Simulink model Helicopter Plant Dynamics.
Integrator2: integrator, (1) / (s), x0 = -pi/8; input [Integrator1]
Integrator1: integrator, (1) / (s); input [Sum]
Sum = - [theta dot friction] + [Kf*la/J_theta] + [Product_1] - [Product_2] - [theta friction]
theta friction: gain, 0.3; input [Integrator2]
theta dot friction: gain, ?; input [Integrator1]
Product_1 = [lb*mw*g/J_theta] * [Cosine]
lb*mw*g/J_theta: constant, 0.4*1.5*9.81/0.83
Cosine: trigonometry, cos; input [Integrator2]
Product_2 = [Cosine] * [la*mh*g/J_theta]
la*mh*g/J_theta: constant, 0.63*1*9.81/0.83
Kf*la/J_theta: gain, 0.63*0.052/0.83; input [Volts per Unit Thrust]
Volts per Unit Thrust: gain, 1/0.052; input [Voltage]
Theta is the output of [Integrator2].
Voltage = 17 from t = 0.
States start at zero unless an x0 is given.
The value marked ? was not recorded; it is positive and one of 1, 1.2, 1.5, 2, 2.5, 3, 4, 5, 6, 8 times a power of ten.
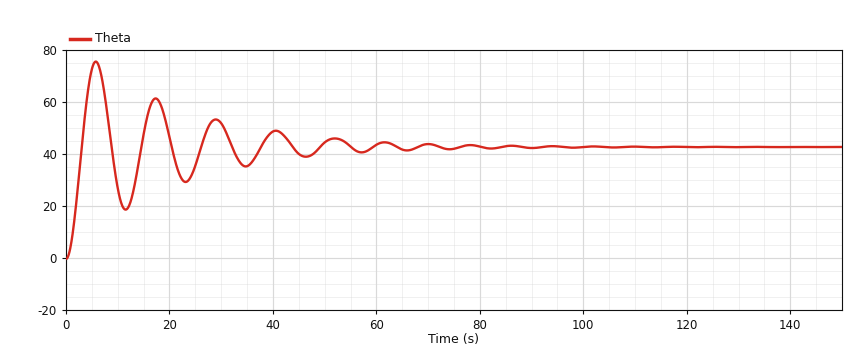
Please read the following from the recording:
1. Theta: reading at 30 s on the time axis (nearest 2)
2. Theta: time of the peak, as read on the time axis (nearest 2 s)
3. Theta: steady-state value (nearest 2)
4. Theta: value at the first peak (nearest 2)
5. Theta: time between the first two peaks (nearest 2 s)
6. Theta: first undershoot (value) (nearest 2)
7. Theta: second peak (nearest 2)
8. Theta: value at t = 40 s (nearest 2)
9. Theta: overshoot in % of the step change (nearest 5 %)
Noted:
52
6 s
42
76
12 s
18
62
48
75 %
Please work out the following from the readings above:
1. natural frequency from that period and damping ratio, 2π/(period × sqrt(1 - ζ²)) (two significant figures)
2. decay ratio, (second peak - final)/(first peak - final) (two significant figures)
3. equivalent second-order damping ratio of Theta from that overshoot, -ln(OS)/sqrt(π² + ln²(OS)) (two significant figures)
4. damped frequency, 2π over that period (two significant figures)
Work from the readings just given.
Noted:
0.53 rad/s
0.59
0.091
0.52 rad/s
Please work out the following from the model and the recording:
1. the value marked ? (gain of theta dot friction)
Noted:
0.1
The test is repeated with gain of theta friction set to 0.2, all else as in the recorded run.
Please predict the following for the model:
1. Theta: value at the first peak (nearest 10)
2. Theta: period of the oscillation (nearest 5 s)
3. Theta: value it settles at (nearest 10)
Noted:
110
15 s
60
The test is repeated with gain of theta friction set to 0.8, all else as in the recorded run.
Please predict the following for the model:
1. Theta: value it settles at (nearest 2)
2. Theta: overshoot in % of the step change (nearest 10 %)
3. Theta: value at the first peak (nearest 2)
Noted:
16
80 %
30
